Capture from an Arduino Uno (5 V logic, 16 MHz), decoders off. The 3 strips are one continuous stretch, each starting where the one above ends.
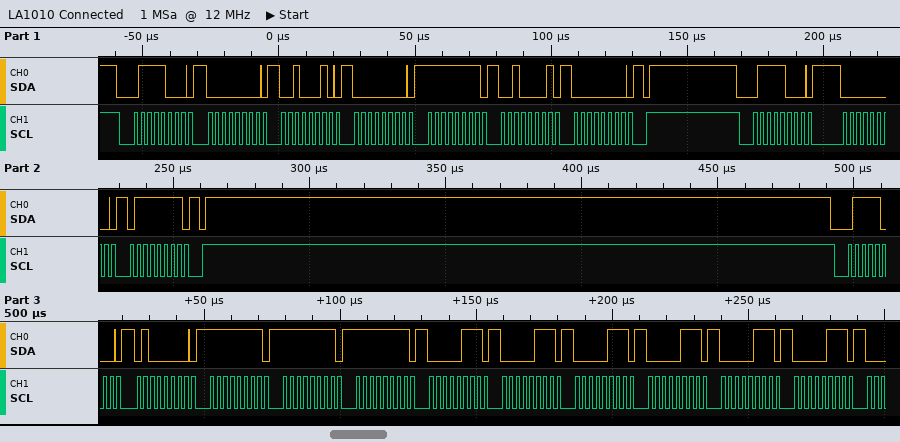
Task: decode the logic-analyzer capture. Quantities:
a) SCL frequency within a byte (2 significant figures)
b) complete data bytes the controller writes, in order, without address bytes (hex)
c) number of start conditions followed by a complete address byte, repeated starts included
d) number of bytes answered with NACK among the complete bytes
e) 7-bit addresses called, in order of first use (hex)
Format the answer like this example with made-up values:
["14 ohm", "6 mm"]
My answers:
["400 kHz", "00 22 00 FF 21 00 00 7F 40 FF FF FF 07 07 07 07 07 07", "3", "0", "0x3C"]
